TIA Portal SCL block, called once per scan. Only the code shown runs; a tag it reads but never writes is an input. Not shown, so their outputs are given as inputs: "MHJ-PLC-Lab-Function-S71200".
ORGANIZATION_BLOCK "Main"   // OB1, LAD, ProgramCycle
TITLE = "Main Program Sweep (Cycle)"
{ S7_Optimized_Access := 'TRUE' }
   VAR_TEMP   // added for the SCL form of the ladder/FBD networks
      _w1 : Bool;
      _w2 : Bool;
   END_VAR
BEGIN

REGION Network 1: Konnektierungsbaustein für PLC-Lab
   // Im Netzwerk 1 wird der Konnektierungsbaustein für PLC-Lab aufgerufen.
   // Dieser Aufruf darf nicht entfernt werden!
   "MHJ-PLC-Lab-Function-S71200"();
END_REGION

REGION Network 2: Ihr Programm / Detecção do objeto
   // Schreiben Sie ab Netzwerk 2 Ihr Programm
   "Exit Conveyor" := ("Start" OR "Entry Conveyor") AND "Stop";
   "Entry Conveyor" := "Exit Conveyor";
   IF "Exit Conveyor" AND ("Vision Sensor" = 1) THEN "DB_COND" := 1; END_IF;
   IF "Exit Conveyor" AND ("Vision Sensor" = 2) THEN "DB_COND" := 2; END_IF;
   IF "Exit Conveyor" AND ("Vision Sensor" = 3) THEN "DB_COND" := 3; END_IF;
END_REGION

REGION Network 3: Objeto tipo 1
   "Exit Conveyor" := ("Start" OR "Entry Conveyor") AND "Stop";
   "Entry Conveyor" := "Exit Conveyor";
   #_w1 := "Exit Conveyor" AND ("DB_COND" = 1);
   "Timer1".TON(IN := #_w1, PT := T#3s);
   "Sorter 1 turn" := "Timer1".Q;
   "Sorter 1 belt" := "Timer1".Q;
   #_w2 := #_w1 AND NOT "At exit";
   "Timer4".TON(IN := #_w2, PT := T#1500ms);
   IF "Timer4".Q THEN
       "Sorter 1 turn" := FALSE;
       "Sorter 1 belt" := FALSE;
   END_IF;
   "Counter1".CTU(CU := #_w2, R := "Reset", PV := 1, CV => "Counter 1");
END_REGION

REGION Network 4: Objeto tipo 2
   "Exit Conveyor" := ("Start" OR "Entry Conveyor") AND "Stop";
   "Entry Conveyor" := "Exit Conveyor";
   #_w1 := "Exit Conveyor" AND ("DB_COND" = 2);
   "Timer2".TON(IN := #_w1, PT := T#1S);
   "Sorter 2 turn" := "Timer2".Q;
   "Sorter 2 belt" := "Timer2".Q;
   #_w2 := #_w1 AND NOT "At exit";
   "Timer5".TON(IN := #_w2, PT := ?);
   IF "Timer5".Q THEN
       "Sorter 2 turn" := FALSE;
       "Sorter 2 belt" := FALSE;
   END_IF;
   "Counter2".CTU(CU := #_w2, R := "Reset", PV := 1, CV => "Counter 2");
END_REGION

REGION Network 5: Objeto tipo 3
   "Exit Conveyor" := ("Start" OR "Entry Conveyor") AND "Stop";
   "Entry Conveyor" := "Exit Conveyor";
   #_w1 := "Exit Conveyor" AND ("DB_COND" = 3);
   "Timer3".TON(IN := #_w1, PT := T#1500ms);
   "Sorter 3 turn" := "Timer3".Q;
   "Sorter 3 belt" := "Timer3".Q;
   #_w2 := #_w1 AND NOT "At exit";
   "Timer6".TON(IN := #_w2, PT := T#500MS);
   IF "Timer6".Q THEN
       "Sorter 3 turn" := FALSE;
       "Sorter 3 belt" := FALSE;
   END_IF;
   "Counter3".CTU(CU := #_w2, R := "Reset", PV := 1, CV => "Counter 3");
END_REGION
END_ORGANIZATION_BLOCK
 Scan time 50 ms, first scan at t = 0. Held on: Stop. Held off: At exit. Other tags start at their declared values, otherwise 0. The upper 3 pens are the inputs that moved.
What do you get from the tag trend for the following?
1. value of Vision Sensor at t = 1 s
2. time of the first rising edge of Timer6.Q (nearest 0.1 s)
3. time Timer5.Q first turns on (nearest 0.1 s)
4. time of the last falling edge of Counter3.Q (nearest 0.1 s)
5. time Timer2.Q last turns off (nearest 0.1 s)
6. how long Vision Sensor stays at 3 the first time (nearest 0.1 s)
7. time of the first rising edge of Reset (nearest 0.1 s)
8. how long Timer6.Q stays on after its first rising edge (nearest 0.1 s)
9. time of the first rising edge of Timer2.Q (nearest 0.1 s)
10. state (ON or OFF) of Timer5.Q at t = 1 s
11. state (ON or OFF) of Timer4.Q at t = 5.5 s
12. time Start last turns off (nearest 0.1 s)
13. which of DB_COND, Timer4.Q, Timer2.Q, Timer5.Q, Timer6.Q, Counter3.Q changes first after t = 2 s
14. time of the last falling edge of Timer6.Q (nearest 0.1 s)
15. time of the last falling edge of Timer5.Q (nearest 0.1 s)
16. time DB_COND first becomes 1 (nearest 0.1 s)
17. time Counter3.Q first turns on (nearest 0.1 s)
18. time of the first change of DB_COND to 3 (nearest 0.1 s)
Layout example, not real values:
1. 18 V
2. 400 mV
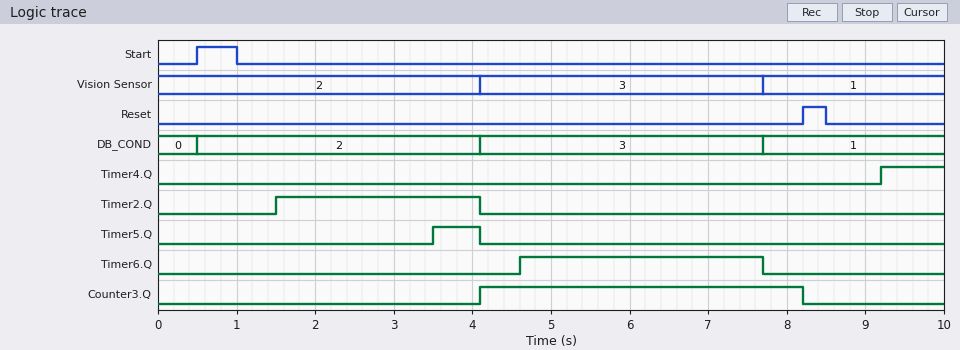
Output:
1. 2
2. 4.6 s
3. 3.5 s
4. 8.2 s
5. 4.1 s
6. 3.6 s
7. 8.2 s
8. 3.1 s
9. 1.5 s
10. OFF
11. OFF
12. 1.0 s
13. Timer5.Q
14. 7.7 s
15. 4.1 s
16. 7.7 s
17. 4.1 s
18. 4.1 s
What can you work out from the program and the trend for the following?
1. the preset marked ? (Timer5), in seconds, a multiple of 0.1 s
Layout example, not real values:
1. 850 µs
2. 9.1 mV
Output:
1. 3.0 s
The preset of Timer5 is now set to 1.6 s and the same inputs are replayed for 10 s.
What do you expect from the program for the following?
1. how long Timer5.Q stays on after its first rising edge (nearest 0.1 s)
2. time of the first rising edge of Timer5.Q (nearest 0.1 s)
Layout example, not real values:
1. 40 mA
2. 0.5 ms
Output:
1. 2.0 s
2. 2.1 s
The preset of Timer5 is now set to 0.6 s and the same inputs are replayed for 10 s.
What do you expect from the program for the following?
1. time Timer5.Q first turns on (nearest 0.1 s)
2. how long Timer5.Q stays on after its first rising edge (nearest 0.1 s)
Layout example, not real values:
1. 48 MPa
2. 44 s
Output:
1. 1.1 s
2. 3.0 s
